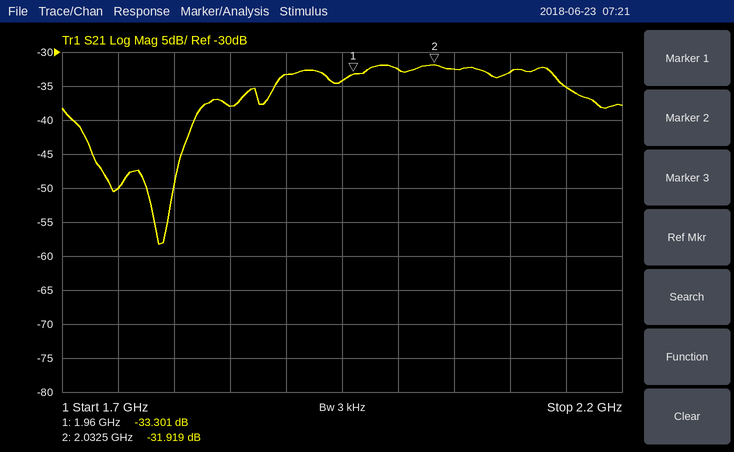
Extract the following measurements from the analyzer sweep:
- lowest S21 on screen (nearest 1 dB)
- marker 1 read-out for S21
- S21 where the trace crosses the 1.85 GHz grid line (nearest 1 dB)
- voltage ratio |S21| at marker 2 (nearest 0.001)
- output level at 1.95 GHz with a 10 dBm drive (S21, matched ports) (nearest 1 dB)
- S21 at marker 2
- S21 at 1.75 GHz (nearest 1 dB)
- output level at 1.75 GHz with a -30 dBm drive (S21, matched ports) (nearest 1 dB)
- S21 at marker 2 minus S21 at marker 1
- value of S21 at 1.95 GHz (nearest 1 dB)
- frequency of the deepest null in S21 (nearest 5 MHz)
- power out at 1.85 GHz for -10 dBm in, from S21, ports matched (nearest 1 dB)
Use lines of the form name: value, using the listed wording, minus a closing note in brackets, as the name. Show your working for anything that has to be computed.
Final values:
lowest S21 on screen: -58 dB
marker 1 read-out for S21: -33.301 dB
S21 where the trace crosses the 1.85 GHz grid line: -38 dB
voltage ratio |S21| at marker 2: 10^(-31.919/20) ≈ 0.025
output level at 1.95 GHz with a 10 dBm drive (S21, matched ports): 10 dBm + (-34 dB) = -24 dBm
S21 at marker 2: -31.919 dB
S21 at 1.75 GHz: -50 dB
output level at 1.75 GHz with a -30 dBm drive (S21, matched ports): -30 dBm + (-50 dB) = -80 dBm
S21 at marker 2 minus S21 at marker 1: -31.919 − (-33.301) = 1.382 dB
value of S21 at 1.95 GHz: -34 dB
frequency of the deepest null in S21: 1.785 GHz
power out at 1.85 GHz for -10 dBm in, from S21, ports matched: -10 dBm + (-38 dB) = -48 dBm
